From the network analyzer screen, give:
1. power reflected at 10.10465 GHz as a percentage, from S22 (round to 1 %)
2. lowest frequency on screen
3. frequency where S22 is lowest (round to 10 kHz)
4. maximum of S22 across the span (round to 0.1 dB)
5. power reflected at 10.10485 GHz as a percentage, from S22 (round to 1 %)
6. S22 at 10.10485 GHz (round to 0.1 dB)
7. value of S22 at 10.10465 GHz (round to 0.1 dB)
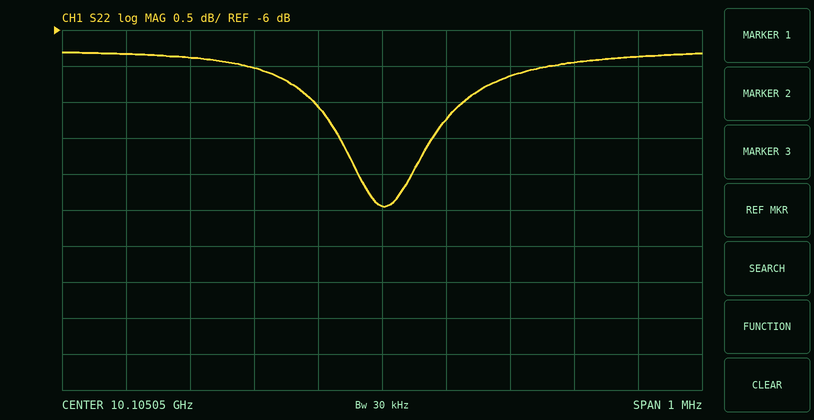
23 %
10.10455 GHz
10.10505 GHz
-6.3 dB
22 %
-6.5 dB
-6.3 dB
